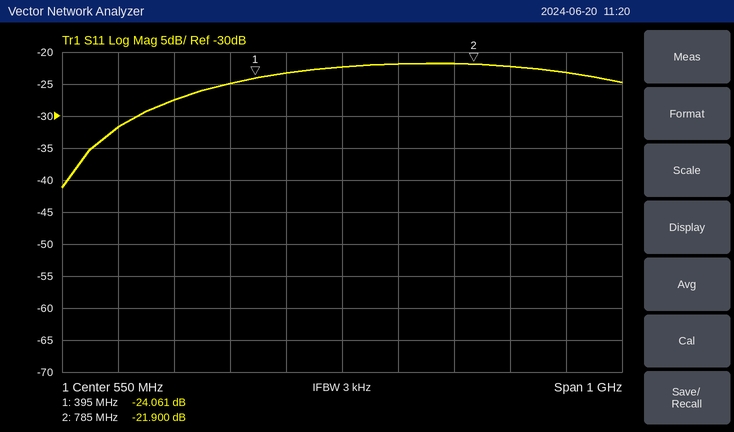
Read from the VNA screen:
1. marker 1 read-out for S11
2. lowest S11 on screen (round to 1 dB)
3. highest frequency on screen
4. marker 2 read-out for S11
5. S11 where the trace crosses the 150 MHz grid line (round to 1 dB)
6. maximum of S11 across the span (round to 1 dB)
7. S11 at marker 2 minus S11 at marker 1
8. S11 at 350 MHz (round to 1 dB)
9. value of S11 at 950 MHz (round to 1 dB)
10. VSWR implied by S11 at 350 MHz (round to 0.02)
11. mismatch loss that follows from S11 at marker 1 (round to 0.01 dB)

-24.061 dB
-41 dB
1.05 GHz
-21.900 dB
-32 dB
-22 dB
2.161 dB
-25 dB
-23 dB
1.12
0.02 dB
